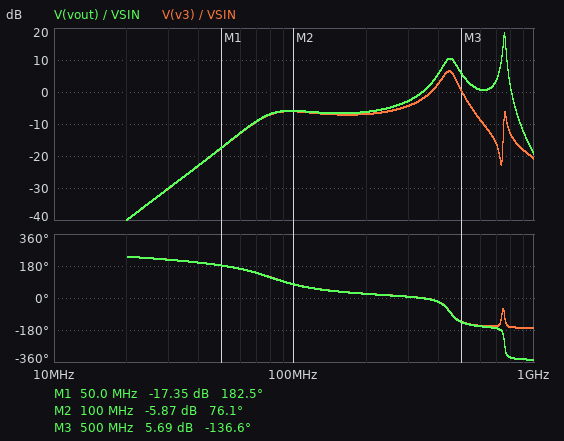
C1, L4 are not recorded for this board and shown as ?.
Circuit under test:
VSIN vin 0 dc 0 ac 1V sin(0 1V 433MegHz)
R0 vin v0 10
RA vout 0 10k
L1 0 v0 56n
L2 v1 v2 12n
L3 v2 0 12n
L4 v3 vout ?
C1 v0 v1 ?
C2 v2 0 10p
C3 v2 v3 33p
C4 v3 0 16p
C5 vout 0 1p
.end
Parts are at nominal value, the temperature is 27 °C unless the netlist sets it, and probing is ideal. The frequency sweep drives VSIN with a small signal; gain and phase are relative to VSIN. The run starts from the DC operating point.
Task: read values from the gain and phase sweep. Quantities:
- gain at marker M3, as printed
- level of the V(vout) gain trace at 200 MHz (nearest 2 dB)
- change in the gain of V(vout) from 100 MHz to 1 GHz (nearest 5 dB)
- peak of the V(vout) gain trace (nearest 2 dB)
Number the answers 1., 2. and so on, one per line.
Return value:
1. 5.69 dB
2. -6 dB
3. -15 dB
4. 18 dB
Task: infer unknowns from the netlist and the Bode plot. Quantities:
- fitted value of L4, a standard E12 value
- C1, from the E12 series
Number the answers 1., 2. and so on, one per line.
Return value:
1. 47 nH
2. 120 pF
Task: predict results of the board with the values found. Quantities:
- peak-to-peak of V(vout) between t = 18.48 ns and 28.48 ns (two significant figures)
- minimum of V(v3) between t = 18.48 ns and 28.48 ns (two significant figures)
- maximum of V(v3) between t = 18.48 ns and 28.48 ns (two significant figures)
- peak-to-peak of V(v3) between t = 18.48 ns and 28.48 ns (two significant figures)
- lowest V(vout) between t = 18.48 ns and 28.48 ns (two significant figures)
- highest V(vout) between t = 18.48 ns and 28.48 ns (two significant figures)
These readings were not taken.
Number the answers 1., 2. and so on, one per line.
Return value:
1. 6.3 V
2. -2.0 V
3. 2.0 V
4. 4.0 V
5. -3.1 V
6. 3.1 V
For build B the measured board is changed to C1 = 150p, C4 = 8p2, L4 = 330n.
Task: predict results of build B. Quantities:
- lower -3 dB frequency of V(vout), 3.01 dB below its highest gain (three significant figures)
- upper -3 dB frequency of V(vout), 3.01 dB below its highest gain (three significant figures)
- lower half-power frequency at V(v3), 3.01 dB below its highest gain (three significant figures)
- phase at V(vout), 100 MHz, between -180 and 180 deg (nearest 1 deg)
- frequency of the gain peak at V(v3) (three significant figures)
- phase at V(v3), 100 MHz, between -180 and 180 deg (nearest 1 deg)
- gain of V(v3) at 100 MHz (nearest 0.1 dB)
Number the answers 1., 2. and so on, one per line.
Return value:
1. 270 MHz
2. 287 MHz
3. 473 MHz
4. 65 deg
5. 507 MHz
6. 66 deg
7. -5.9 dB
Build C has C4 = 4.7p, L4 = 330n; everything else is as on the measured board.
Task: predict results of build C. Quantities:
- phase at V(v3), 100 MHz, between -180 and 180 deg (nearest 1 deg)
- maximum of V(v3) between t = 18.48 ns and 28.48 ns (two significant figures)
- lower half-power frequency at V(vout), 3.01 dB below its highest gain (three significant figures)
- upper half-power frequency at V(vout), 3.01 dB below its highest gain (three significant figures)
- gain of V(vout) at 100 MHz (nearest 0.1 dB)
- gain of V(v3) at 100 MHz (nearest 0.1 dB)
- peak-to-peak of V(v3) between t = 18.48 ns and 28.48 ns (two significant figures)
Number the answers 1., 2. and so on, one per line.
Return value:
1. 78 deg
2. 1.1 V
3. 270 MHz
4. 287 MHz
5. -2.8 dB
6. -4.0 dB
7. 2.2 V
